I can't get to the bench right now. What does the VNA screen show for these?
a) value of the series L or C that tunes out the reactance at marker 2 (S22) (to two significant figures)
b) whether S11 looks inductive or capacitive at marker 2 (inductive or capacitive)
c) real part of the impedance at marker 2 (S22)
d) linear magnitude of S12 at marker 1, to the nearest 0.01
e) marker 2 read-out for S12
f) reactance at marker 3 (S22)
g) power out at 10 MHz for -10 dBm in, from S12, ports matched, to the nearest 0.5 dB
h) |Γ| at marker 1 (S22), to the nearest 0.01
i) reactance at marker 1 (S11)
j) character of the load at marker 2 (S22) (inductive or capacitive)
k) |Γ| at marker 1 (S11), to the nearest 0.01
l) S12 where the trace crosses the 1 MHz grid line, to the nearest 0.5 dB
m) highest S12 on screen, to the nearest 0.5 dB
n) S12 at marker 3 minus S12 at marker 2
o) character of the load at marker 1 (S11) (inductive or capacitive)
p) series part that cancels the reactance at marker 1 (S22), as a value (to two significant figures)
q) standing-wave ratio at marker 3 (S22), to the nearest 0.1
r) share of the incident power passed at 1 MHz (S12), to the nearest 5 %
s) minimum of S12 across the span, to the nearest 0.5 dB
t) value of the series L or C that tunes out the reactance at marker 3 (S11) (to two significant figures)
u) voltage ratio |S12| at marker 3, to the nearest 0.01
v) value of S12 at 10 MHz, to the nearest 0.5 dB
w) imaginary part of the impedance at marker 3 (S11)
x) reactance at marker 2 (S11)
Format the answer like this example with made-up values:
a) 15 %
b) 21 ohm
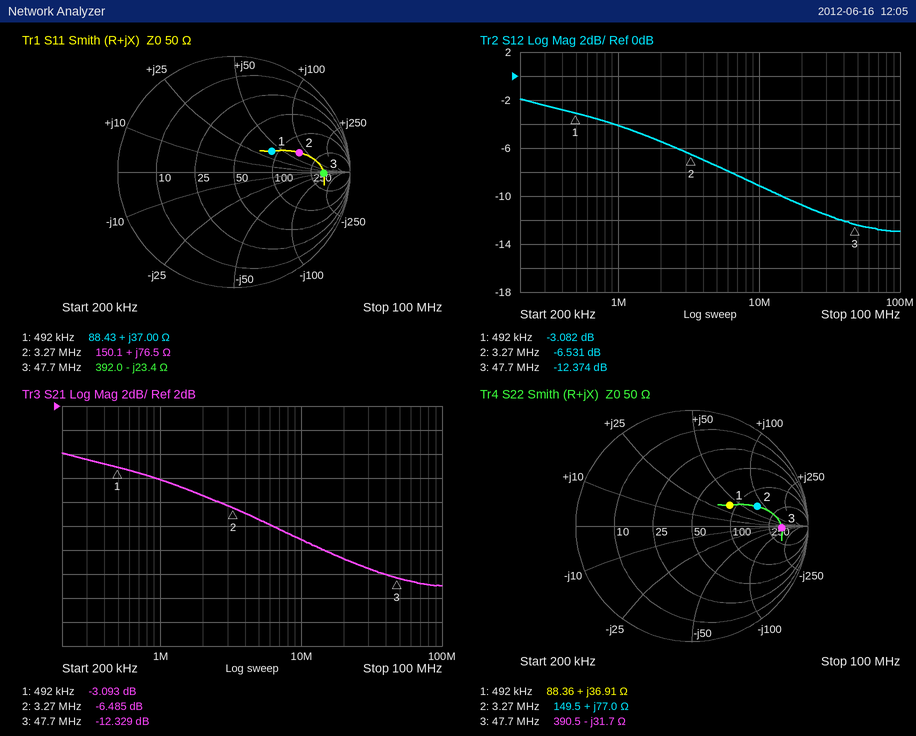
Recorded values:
a) 630 pF
b) inductive
c) 149.5 Ω
d) 0.70
e) -6.531 dB
f) -31.7 Ω
g) -19.0 dBm
h) 0.37
i) +37.00 Ω
j) inductive
k) 0.37
l) -4.0 dB
m) -2.0 dB
n) -5.843 dB
o) inductive
p) 8.8 nF
q) 7.9
r) 40 %
s) -13.0 dB
t) 78 nH
u) 0.24
v) -9.0 dB
w) -23.4 Ω
x) +76.5 Ω
